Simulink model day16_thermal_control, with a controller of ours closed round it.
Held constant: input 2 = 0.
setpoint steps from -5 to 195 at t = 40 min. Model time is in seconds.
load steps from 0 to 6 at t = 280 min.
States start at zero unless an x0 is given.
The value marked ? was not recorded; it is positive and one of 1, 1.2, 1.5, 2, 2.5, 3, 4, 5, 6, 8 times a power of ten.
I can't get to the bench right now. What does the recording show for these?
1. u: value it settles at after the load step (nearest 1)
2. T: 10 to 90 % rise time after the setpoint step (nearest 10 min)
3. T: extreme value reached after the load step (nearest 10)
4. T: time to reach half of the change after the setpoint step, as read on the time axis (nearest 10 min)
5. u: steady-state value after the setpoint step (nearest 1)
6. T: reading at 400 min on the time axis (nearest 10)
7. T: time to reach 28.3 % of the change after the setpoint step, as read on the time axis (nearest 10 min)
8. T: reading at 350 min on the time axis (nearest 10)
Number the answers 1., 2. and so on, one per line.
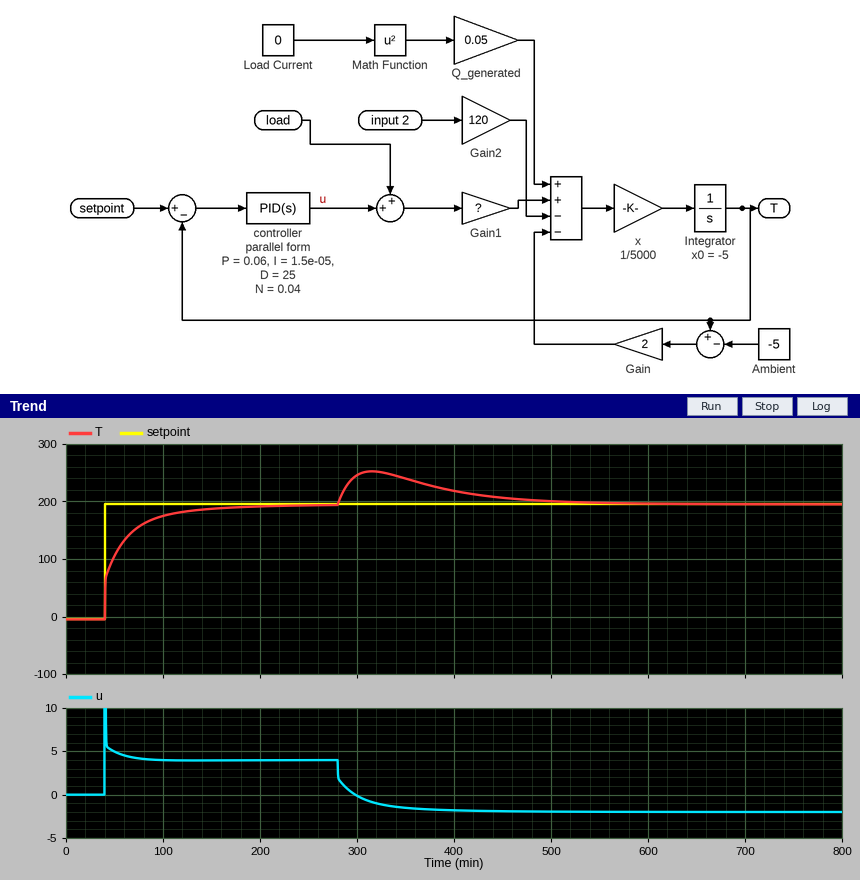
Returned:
1. -2
2. 60 min
3. 250
4. 50 min
5. 4
6. 220
7. 40 min
8. 240
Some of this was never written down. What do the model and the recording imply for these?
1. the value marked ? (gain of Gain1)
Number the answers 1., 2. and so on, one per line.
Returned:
1. 100
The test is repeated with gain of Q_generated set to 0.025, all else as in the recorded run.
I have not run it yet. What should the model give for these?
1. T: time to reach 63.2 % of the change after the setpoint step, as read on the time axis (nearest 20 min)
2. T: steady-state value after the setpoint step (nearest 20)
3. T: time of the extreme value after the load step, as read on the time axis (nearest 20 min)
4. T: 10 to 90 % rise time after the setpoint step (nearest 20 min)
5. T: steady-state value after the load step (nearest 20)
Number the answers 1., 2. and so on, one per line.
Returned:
1. 60 min
2. 200
3. 320 min
4. 60 min
5. 200
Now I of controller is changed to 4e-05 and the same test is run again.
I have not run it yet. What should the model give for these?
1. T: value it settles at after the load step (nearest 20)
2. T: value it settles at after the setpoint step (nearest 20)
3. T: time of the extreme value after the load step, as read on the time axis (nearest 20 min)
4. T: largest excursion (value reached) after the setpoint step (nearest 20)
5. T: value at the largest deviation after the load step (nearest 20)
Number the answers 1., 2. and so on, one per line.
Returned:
1. 200
2. 200
3. 300 min
4. 200
5. 240
